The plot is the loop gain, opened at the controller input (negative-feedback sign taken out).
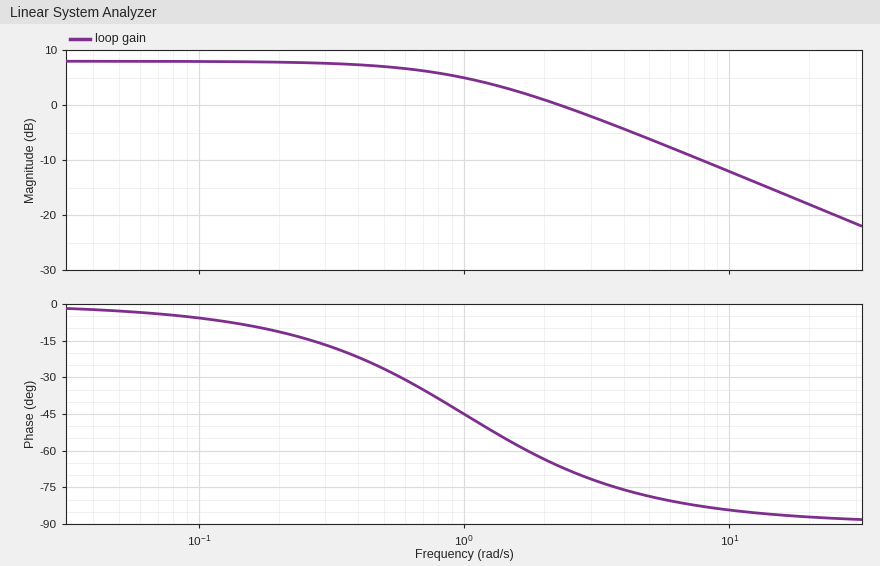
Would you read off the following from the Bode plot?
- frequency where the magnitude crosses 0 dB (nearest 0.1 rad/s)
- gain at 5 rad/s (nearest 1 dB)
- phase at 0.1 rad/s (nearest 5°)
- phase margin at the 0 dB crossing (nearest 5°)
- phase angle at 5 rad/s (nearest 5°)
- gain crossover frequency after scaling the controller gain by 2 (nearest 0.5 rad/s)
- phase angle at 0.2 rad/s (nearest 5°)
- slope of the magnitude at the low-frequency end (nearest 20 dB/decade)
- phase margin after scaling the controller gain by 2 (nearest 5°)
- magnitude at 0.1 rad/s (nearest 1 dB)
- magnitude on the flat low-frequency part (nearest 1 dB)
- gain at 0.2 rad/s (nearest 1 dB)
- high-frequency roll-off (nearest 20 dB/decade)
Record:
2.3 rad/s
-6 dB
-5°
115°
-80°
5.0 rad/s
-10°
0 dB/decade
100°
8 dB
8 dB
8 dB
-20 dB/decade
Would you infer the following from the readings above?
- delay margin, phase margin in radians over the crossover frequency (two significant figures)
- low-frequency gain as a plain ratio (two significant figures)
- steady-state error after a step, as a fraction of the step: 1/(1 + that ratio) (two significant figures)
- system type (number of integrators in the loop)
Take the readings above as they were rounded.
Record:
0.87 s
2.5
0.29
0
